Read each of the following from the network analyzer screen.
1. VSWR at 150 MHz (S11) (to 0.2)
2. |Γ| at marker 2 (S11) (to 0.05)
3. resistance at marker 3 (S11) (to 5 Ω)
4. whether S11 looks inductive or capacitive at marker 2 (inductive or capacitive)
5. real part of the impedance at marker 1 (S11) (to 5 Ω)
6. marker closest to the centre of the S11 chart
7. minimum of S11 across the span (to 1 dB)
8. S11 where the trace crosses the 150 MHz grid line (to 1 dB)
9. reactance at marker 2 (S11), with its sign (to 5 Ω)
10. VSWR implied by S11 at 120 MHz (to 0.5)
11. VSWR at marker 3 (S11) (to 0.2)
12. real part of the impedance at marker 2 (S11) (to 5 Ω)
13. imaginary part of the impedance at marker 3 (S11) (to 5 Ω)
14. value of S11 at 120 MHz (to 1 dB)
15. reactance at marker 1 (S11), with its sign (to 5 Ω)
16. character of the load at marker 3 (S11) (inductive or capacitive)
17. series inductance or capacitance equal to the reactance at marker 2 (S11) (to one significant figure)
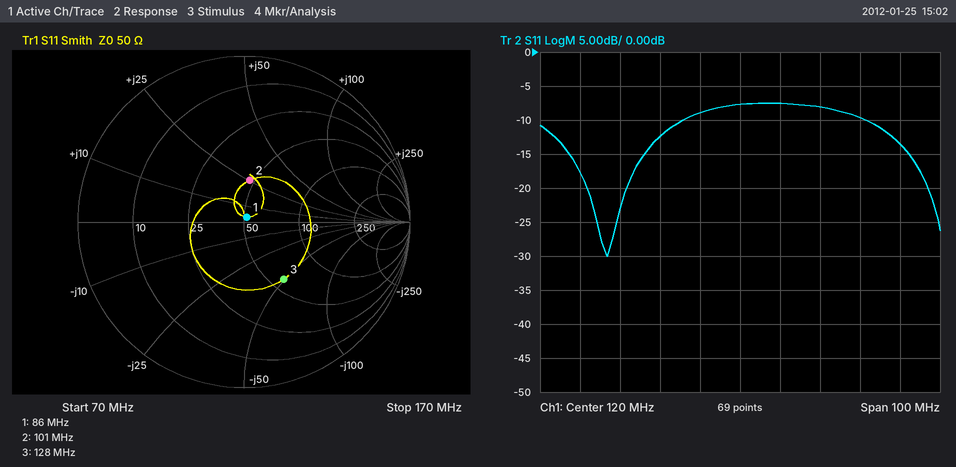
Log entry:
2.0
0.25
60 Ω
inductive
50 Ω
marker 1
-30 dB
-10 dB
+25 Ω
2.5
2.4
45 Ω
-50 Ω
-8 dB
+5 Ω
capacitive
40 nH
